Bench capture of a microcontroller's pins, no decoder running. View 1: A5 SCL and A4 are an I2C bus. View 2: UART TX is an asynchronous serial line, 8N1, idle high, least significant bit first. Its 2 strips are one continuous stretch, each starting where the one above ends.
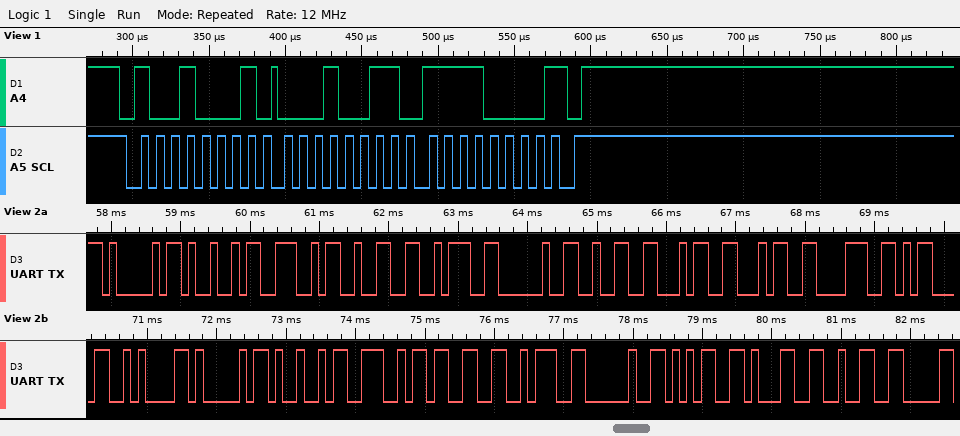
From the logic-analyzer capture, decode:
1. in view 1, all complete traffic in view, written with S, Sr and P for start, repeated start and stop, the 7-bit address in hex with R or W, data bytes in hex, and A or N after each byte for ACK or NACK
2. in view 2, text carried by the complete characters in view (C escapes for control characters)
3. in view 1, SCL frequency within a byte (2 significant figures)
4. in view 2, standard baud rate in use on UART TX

S 48R A 13 A F0 N P
"AIN2: 2448\r\nAIN3: 512"
100 kHz
9600 baud
